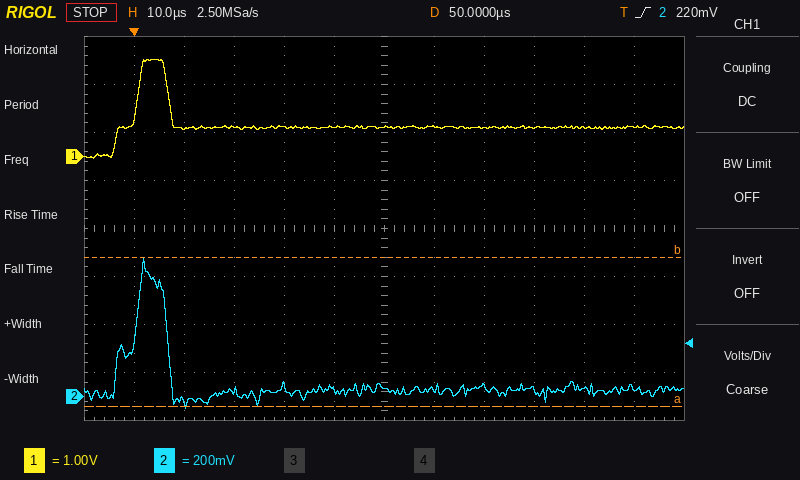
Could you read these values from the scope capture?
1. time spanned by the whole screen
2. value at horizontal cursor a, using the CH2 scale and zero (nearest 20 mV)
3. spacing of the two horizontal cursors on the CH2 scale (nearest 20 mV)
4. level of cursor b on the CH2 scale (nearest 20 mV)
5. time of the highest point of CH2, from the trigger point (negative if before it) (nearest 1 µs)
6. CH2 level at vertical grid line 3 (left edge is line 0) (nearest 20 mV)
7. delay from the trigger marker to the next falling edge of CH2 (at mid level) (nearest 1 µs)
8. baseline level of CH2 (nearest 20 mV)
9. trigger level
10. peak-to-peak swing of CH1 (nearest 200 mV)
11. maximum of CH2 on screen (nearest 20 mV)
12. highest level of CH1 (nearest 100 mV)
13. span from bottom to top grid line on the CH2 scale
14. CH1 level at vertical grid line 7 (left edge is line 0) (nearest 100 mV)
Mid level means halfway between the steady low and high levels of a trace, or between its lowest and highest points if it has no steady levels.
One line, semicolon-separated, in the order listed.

120 µs; -40 mV; 620 mV; 580 mV; +2 µs; 20 mV; 7 µs; 20 mV; 220 mV; 2.0 V; 580 mV; 2.0 V; 1.6 V; 600 mV
